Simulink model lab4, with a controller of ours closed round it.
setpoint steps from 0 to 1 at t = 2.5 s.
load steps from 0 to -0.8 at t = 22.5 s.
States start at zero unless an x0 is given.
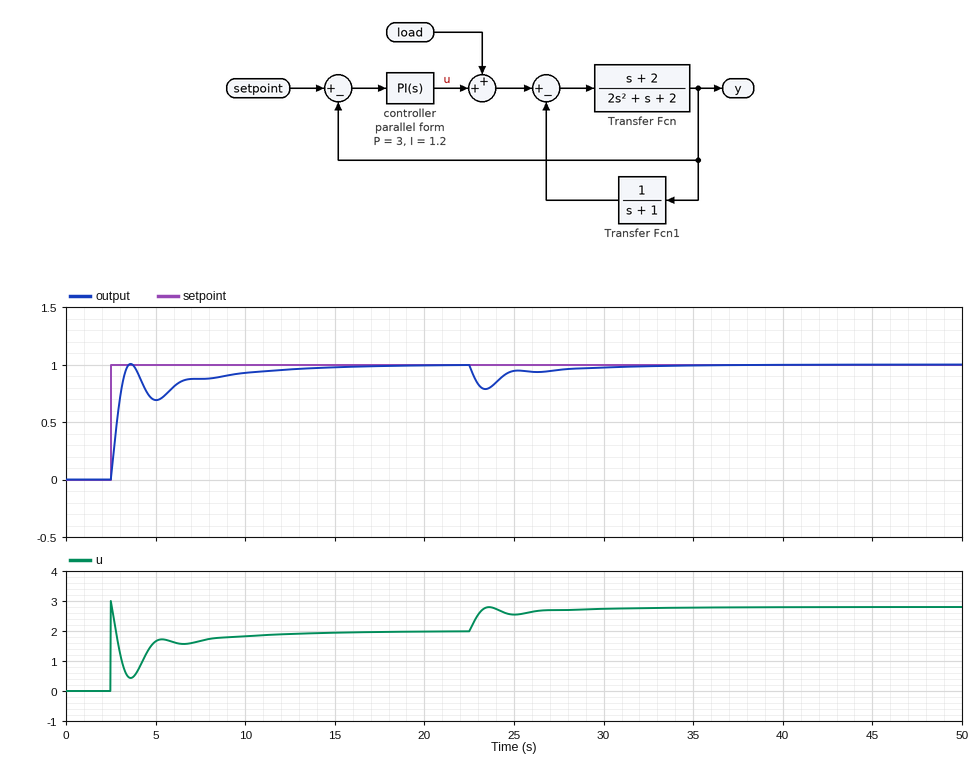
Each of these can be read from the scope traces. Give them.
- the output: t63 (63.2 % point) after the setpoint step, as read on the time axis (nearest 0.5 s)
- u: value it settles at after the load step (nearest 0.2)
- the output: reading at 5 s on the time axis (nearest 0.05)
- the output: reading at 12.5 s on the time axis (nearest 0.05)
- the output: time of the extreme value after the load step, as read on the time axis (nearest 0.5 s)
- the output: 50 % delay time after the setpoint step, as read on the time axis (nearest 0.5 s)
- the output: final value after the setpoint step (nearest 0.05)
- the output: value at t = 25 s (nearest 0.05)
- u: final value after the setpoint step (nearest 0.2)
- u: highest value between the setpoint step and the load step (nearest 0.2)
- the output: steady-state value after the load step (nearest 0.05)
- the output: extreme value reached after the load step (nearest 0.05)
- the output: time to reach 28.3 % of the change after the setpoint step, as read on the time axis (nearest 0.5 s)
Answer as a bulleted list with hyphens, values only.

- 3.0 s
- 2.8
- 0.70
- 0.95
- 23.5 s
- 3.0 s
- 1.00
- 0.95
- 2.0
- 3.0
- 1.00
- 0.80
- 2.5 s
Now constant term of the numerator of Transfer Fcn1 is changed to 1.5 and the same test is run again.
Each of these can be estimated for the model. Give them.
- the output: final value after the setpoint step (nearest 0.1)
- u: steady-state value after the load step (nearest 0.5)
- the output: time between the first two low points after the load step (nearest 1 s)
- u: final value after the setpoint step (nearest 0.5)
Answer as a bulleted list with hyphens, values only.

- 1.0
- 3.5
- 3 s
- 2.5
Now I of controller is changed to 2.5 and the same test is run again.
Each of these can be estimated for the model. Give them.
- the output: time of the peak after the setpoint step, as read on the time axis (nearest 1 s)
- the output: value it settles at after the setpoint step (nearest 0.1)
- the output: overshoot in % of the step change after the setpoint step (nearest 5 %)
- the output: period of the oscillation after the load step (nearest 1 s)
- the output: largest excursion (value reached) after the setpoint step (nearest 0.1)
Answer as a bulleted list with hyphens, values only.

- 4 s
- 1.0
- 10 %
- 3 s
- 1.1
